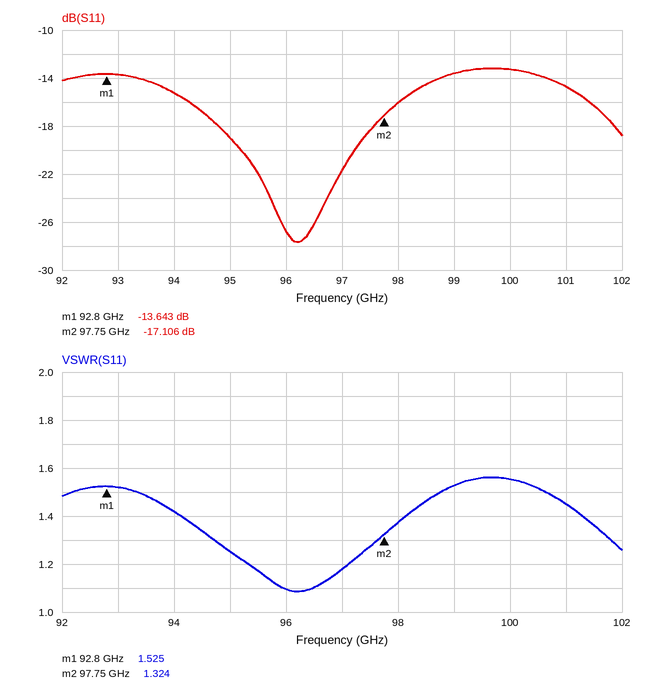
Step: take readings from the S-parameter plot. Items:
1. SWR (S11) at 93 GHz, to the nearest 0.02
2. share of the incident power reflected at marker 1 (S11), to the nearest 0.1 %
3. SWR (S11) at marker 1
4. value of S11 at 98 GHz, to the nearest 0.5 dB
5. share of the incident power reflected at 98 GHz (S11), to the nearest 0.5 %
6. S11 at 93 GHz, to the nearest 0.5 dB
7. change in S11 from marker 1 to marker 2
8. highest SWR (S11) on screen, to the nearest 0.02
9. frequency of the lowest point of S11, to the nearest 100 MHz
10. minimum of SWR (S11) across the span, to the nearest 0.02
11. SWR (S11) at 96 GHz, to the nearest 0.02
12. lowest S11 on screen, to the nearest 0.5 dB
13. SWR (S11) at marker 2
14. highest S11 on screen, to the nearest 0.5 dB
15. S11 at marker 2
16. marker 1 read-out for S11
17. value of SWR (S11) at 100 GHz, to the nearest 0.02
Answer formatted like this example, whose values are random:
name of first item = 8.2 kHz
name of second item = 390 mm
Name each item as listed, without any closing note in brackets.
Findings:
SWR (S11) at 93 GHz, to the nearest 0.02 = 1.52
share of the incident power reflected at marker 1 (S11), to the nearest 0.1 % = 4.3 %
SWR (S11) at marker 1 = 1.525
value of S11 at 98 GHz, to the nearest 0.5 dB = -16.0 dB
share of the incident power reflected at 98 GHz (S11), to the nearest 0.5 % = 2.5 %
S11 at 93 GHz, to the nearest 0.5 dB = -13.5 dB
change in S11 from marker 1 to marker 2 = -3.463 dB
highest SWR (S11) on screen, to the nearest 0.02 = 1.56
frequency of the lowest point of S11, to the nearest 100 MHz = 96.2 GHz
minimum of SWR (S11) across the span, to the nearest 0.02 = 1.08
SWR (S11) at 96 GHz, to the nearest 0.02 = 1.10
lowest S11 on screen, to the nearest 0.5 dB = -27.5 dB
SWR (S11) at marker 2 = 1.324
highest S11 on screen, to the nearest 0.5 dB = -13.0 dB
S11 at marker 2 = -17.106 dB
marker 1 read-out for S11 = -13.643 dB
value of SWR (S11) at 100 GHz, to the nearest 0.02 = 1.56
